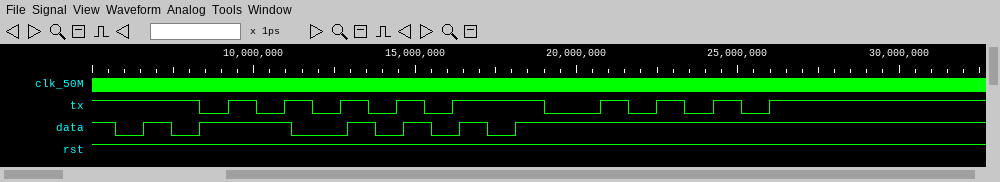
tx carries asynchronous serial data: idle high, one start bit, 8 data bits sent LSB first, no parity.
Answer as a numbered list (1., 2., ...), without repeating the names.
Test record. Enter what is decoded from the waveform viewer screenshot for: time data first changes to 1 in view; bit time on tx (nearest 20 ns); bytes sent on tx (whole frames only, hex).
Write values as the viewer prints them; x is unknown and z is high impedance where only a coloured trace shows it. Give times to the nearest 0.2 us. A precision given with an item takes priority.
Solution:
1. 6.6 us
2. 880 ns
3. 55, AA
